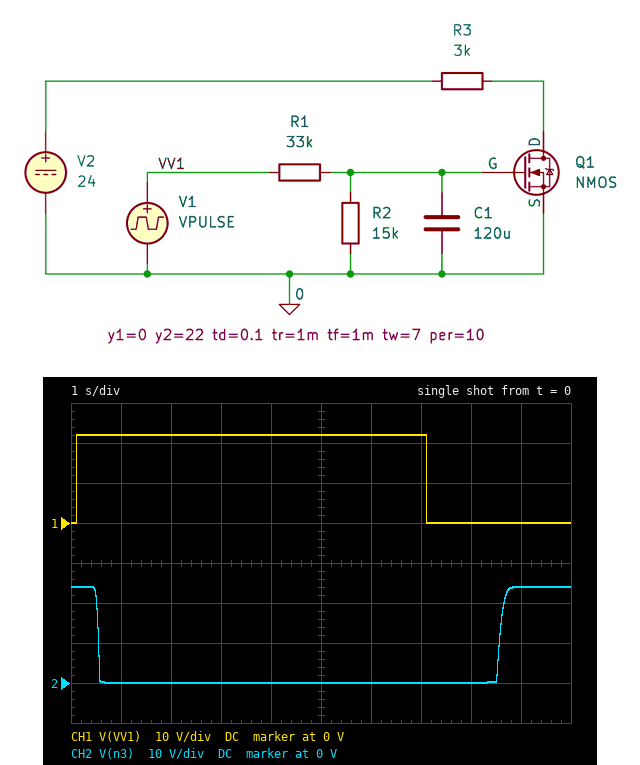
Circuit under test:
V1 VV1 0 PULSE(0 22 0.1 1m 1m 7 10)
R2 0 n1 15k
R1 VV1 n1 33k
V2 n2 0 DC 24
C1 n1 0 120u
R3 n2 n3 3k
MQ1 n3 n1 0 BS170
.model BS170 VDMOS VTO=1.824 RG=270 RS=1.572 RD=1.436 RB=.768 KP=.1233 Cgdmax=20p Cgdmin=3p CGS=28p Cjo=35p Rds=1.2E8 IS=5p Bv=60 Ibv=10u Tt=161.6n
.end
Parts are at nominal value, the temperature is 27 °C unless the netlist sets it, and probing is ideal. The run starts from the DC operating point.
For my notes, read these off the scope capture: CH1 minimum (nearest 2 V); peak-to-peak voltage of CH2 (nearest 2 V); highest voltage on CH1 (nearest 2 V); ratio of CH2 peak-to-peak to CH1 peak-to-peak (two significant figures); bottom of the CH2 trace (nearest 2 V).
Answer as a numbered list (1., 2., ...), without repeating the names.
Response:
1. 0 V
2. 24 V
3. 22 V
4. 1.1
5. 0 V
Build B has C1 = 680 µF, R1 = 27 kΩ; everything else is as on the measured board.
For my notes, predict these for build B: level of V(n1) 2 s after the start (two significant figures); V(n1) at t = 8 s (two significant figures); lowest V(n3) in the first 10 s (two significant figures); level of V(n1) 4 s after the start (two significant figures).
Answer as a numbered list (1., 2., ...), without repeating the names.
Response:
1. 2.0 V
2. 4.5 V
3. 44 mV
4. 3.5 V
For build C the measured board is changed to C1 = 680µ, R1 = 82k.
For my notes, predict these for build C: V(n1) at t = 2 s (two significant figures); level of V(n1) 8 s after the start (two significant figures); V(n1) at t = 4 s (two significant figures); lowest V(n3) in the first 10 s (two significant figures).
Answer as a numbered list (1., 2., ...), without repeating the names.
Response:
1. 670 mV
2. 1.7 V
3. 1.2 V
4. 22 V
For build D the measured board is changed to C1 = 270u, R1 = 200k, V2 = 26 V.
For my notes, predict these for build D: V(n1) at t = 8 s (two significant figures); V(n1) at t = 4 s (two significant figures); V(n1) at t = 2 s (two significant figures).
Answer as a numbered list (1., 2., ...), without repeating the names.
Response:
1. 1.0 V
2. 990 mV
3. 610 mV
